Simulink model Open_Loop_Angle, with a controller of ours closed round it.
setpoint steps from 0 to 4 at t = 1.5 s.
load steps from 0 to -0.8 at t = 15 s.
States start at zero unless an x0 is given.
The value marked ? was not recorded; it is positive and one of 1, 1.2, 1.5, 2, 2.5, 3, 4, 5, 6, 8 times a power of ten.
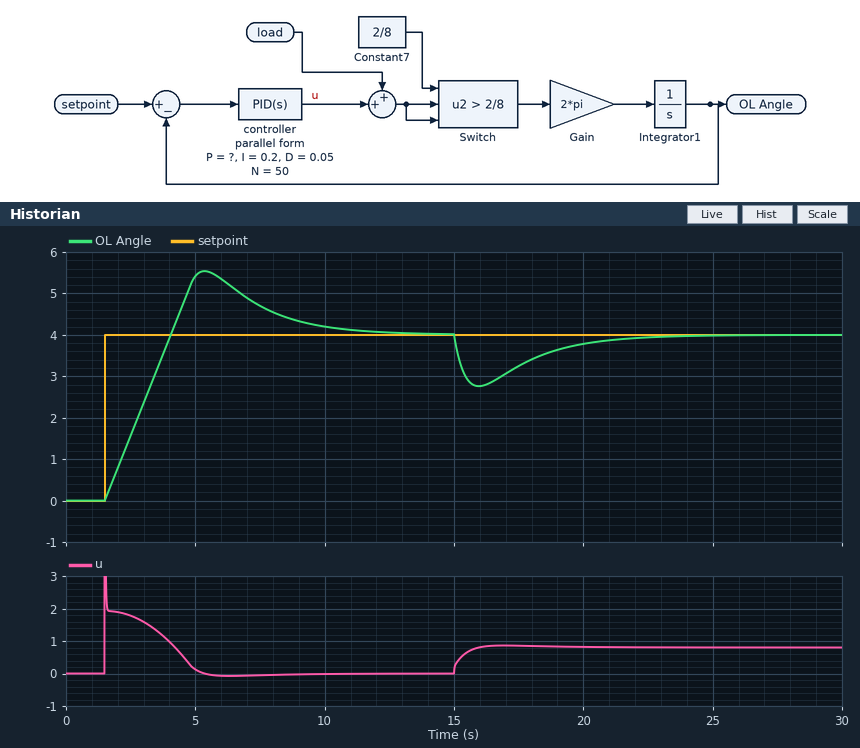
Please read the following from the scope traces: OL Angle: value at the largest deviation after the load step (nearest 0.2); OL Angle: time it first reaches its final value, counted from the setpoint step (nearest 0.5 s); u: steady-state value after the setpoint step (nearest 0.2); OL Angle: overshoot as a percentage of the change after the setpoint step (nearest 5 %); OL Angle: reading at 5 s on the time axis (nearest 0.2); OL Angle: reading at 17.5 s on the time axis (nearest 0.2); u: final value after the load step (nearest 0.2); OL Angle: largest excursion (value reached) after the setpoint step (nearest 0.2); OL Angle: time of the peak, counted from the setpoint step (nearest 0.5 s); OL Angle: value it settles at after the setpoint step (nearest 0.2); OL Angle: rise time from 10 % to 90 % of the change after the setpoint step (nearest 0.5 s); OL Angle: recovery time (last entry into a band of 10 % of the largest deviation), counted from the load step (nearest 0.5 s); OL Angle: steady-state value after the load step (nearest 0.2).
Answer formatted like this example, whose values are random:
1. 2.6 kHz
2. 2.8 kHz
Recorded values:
1. 2.8
2. 2.5 s
3. 0.0
4. 40 %
5. 5.4
6. 3.2
7. 0.8
8. 5.6
9. 4.0 s
10. 4.0
11. 2.0 s
12. 6.0 s
13. 4.0
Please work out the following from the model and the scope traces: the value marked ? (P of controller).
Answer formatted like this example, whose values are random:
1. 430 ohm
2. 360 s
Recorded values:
1. 0.5
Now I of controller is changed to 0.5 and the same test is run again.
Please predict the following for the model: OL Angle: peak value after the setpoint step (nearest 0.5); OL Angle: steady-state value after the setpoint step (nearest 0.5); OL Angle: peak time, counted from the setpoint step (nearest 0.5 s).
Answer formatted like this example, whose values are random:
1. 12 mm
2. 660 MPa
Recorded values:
1. 6.5
2. 4.0
3. 4.5 s
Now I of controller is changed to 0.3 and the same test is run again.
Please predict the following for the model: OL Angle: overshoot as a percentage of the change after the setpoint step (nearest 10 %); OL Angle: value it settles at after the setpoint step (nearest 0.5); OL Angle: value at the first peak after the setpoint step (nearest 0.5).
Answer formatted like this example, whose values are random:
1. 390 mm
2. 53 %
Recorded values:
1. 50 %
2. 4.0
3. 6.0
